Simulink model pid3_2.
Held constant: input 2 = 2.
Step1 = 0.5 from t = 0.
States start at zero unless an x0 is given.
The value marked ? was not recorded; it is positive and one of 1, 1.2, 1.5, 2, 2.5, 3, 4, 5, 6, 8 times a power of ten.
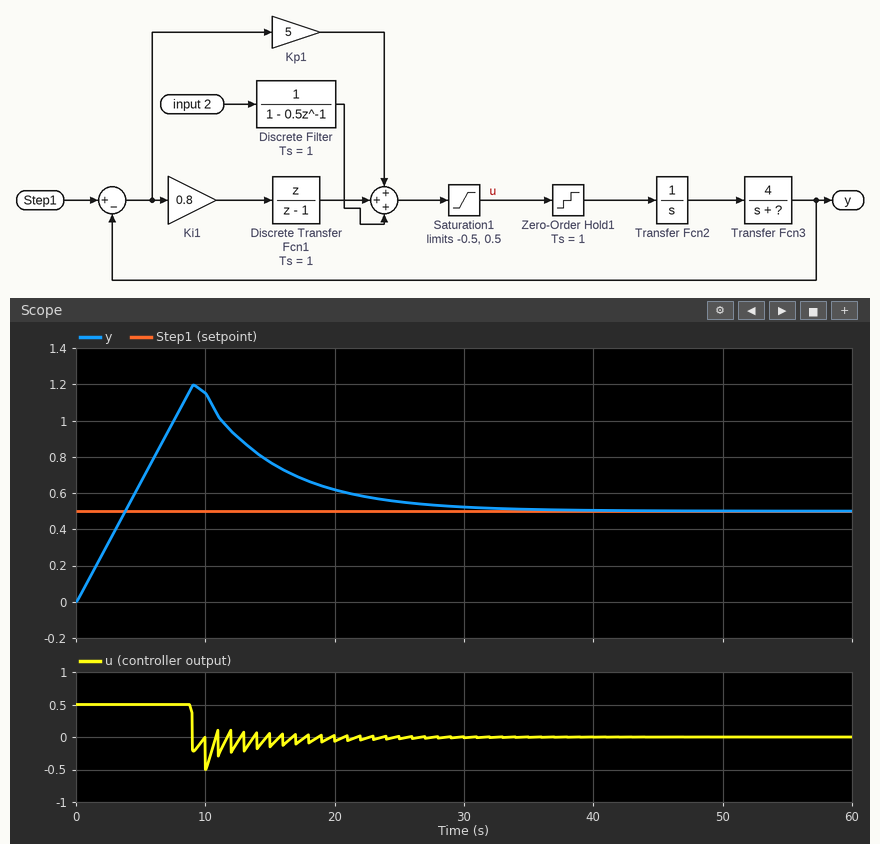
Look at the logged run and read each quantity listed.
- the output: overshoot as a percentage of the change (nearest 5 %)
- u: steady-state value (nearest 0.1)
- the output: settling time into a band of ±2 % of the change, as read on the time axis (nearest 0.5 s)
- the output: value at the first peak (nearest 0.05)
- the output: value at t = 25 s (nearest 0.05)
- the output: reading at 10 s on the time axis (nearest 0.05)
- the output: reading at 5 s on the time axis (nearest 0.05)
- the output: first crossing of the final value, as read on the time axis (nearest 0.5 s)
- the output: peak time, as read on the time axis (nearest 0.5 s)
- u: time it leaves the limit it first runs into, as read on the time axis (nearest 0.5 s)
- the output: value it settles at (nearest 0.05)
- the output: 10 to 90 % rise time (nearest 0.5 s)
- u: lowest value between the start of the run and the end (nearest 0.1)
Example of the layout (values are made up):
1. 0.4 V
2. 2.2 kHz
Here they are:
1. 140 %
2. 0.0
3. 35.0 s
4. 1.20
5. 0.55
6. 1.15
7. 0.65
8. 4.0 s
9. 9.0 s
10. 9.0 s
11. 0.50
12. 3.0 s
13. -0.5
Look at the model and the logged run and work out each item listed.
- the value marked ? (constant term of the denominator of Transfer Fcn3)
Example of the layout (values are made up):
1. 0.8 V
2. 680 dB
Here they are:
1. 15
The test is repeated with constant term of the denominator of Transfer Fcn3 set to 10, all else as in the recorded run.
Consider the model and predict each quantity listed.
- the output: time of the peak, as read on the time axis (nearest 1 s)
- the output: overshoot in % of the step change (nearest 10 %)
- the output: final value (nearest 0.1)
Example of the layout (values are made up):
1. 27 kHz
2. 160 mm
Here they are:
1. 7 s
2. 150 %
3. 0.5
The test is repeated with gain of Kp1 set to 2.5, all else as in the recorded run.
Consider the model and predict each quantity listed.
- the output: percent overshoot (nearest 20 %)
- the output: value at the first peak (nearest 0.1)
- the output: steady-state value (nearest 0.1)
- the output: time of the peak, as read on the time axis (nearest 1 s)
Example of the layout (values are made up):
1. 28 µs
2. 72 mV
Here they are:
1. 200 %
2. 1.5
3. 0.5
4. 11 s
